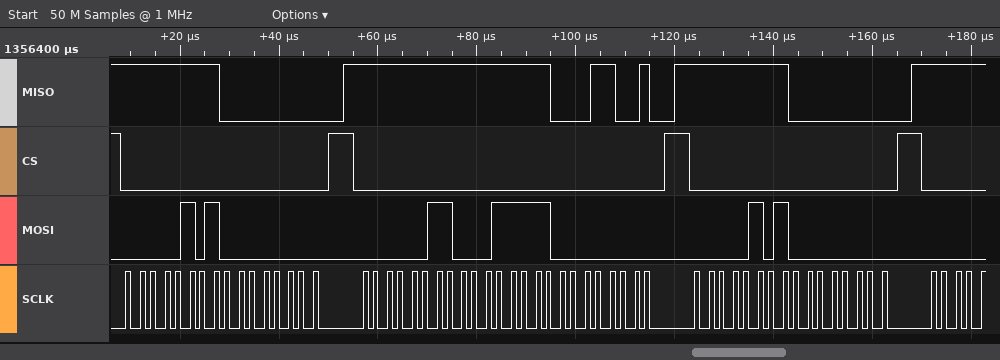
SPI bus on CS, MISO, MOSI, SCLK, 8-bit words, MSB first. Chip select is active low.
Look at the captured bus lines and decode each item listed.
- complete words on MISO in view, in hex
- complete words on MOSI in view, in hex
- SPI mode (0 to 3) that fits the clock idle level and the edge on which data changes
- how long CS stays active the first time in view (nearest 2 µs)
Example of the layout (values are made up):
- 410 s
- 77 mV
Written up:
- FF, 00, FF, FF, 19, FF, 00
- 05, 00, 03, 1F, 00, 05, 00
- 0
- 42 µs
